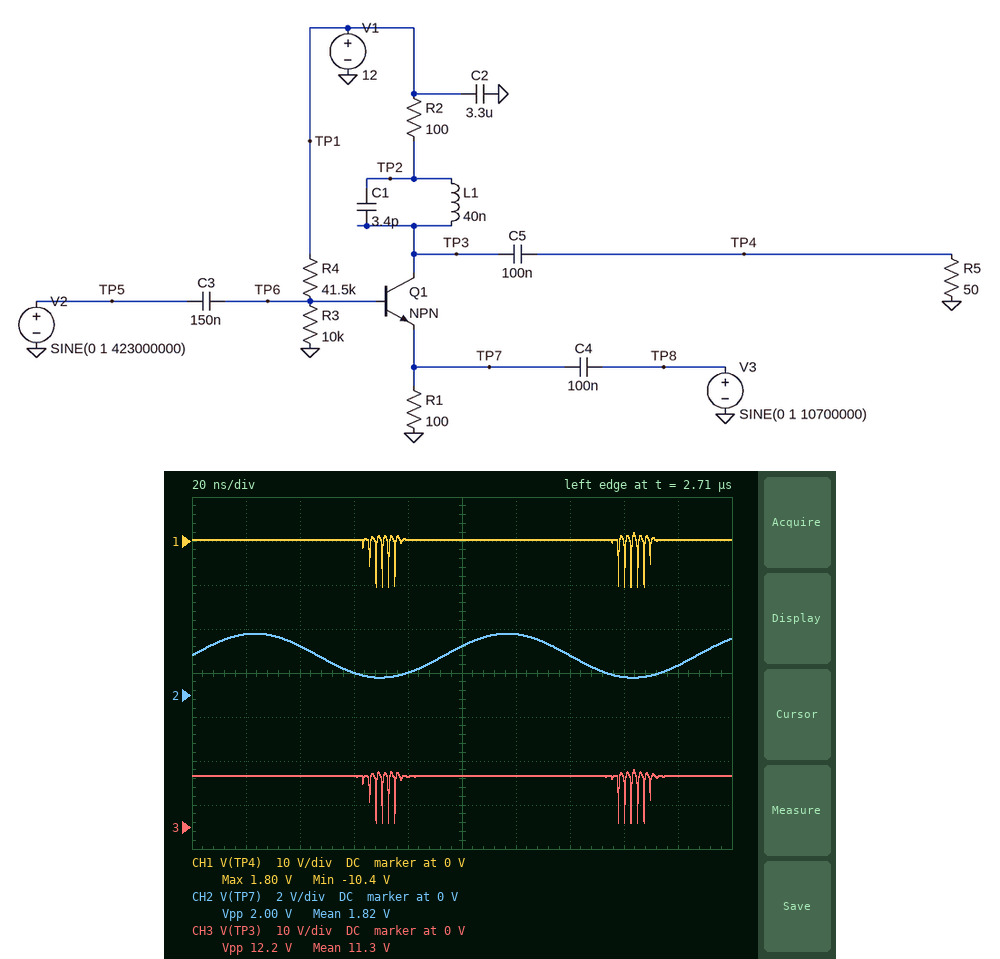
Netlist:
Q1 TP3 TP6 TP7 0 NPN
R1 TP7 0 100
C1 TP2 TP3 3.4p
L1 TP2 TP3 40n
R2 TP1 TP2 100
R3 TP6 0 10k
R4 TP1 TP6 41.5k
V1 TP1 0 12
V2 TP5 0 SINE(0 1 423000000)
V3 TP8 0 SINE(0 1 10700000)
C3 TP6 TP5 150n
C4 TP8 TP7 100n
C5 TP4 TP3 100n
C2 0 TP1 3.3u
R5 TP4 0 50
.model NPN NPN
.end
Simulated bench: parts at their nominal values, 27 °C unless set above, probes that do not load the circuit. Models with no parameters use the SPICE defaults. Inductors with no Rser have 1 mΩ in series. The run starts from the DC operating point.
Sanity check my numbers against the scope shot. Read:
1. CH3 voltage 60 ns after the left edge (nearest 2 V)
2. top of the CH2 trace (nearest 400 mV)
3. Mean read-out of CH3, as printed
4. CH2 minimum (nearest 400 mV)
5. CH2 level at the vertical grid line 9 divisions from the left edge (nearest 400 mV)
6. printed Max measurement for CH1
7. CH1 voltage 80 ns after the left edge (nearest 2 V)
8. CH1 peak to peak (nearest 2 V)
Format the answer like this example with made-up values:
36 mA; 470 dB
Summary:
12 V; 2.8 V; 11.3 V; 800 mV; 1.2 V; 1.80 V; 0 V; 12 V
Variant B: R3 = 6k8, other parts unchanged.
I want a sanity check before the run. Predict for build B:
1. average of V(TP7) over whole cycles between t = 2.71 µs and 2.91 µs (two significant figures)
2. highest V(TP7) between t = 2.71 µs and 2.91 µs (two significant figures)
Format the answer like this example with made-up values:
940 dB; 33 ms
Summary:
1.5 V; 2.5 V
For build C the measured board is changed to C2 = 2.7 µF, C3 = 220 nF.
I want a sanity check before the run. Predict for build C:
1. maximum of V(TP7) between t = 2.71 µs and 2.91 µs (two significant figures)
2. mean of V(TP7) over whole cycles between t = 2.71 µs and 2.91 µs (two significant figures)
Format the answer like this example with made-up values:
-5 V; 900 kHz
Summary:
3.0 V; 2.0 V
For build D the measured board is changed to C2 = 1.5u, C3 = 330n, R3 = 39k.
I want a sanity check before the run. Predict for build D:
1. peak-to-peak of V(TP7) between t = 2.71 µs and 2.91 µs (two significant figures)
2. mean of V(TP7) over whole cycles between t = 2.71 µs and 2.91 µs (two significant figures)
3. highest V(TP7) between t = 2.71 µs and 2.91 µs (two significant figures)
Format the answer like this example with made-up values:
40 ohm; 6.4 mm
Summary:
2.0 V; 2.9 V; 3.9 V
